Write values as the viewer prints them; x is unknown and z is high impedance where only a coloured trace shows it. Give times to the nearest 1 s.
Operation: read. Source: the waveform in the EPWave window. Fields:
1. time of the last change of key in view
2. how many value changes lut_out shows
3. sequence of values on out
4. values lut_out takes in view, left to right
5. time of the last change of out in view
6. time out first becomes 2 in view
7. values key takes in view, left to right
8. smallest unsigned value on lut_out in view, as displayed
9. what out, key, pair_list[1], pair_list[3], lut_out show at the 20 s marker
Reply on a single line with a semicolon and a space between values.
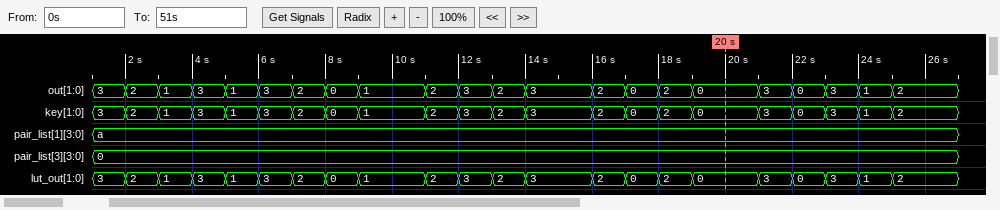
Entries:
25 s; 21; 3, 2, 1, 3, 1, 3, 2, 0, 1, 2, 3, 2, 3, 2, 0, 2, 0, 3, 0, 3, 1, 2; 3, 2, 1, 3, 1, 3, 2, 0, 1, 2, 3, 2, 3, 2, 0, 2, 0, 3, 0, 3, 1, 2; 25 s; 2 s; 3, 2, 1, 3, 1, 3, 2, 0, 1, 2, 3, 2, 3, 2, 0, 2, 0, 3, 0, 3, 1, 2; 0; out=0, key=0, pair_list[1]=a, pair_list[3]=0, lut_out=0
